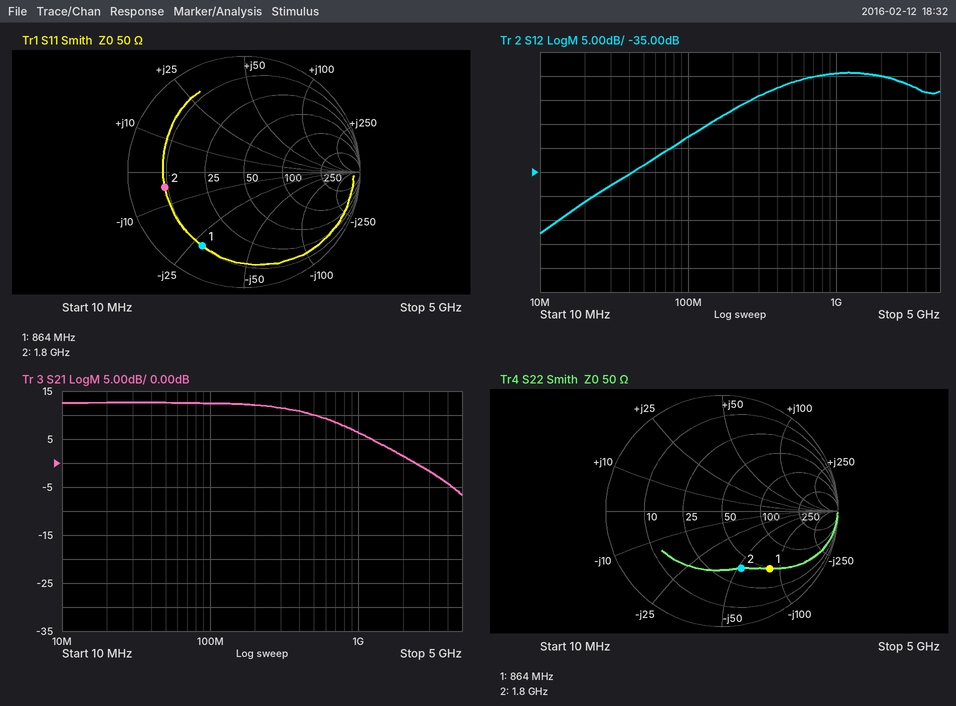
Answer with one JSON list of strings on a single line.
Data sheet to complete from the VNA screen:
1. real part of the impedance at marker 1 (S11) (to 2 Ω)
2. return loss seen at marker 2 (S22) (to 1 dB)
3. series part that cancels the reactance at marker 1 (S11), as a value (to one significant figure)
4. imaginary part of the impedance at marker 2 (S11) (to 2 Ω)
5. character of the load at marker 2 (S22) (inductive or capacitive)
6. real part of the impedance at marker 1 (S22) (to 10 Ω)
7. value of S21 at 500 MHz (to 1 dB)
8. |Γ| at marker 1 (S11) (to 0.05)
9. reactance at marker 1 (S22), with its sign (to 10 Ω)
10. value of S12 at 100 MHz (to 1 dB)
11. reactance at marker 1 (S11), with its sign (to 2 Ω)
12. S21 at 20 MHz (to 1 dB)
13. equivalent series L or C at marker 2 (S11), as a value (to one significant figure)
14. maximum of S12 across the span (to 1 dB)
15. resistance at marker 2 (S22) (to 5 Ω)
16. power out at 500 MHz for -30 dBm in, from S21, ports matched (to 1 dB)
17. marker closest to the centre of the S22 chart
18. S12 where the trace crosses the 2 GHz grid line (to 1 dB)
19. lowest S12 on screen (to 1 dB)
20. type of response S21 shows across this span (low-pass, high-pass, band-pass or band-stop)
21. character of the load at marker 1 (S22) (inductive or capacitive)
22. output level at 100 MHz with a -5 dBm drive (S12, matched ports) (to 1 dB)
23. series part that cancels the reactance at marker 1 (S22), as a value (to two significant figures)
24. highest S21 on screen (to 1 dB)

["10 Ω", "6 dB", "5 nH", "-4 Ω", "capacitive", "50 Ω", "10 dB", "0.75", "-80 Ω", "-28 dB", "-28 Ω", "13 dB", "20 pF", "-14 dB", "40 Ω", "-20 dBm", "marker 2", "-15 dB", "-48 dB", "low-pass", "capacitive", "-33 dBm", "15 nH", "13 dB"]
